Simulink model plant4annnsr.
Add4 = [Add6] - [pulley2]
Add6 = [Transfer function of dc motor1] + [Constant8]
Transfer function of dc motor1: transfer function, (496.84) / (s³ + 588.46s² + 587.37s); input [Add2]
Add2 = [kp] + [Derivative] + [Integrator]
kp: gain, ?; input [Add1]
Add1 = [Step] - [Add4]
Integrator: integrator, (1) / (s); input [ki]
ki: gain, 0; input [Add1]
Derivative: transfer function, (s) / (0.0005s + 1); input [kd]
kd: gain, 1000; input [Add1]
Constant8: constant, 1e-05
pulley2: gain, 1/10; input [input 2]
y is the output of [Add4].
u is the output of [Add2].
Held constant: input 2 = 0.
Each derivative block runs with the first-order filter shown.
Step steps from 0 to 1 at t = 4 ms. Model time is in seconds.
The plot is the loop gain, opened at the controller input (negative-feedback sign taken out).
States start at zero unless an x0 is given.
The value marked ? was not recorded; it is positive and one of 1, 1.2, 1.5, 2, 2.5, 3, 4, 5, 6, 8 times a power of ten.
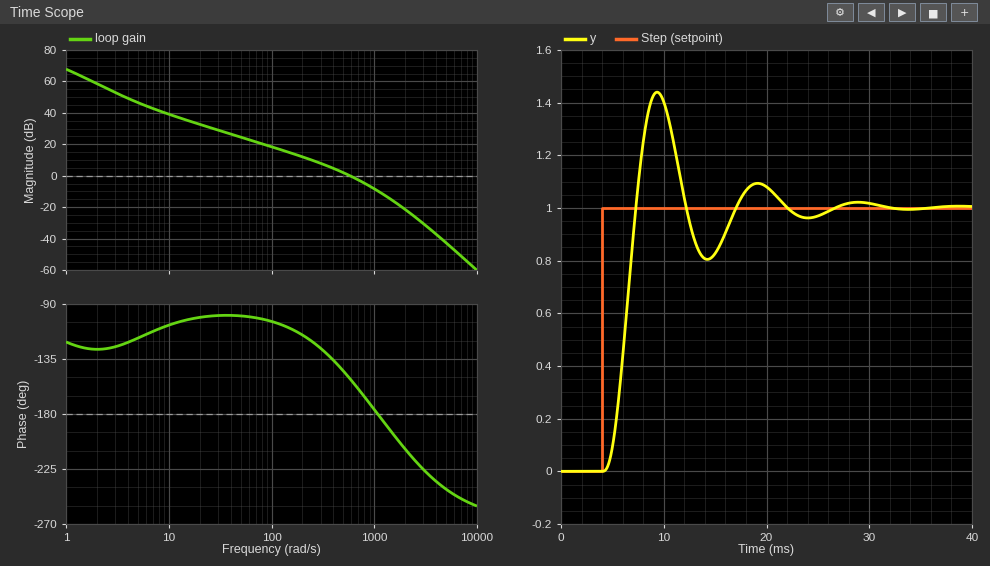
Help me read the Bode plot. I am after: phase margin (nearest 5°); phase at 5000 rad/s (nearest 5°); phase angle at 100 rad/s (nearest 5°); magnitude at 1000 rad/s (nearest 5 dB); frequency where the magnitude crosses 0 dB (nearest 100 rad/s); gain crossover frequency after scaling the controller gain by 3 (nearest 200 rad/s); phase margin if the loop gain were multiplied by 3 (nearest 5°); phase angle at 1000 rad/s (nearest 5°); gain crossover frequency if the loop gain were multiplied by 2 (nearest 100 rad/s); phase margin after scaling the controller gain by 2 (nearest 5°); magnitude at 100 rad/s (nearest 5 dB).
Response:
30°
-240°
-105°
-10 dB
600 rad/s
1000 rad/s
0°
-175°
900 rad/s
10°
20 dB
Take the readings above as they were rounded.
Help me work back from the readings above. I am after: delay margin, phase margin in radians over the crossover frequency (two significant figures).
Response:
0.00087 s
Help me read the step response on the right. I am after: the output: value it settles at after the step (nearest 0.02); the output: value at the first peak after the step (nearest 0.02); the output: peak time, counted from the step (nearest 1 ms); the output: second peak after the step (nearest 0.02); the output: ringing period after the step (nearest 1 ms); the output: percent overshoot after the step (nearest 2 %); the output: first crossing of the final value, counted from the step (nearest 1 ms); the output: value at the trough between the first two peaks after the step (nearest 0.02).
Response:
1.00
1.44
5 ms
1.10
10 ms
44 %
3 ms
0.80
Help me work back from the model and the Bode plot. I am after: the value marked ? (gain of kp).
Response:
4000
